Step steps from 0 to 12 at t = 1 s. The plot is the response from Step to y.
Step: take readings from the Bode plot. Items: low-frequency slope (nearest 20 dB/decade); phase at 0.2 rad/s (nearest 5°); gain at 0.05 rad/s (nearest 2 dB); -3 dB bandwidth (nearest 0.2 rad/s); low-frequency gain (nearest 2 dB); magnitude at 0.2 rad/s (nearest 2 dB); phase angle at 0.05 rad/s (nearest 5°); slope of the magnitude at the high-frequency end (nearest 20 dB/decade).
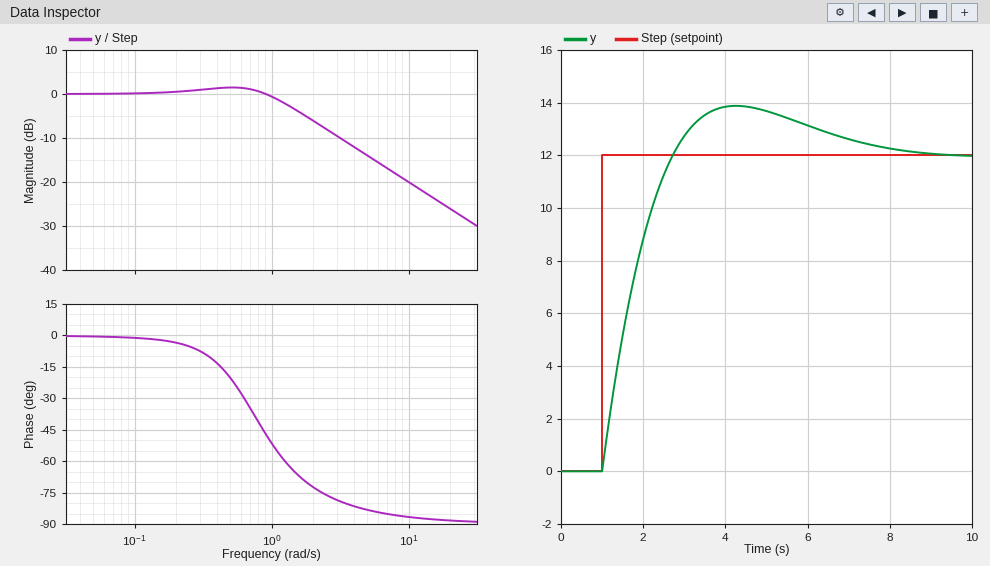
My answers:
0 dB/decade
-5°
0 dB
1.4 rad/s
0 dB
0 dB
0°
-20 dB/decade
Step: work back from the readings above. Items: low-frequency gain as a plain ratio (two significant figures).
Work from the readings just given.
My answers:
1.0
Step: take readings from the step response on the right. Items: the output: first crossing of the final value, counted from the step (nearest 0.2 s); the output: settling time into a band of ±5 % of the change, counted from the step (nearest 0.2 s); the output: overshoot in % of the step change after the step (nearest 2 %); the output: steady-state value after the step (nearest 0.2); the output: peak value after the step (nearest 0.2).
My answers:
1.8 s
6.0 s
16 %
12.0
13.8
